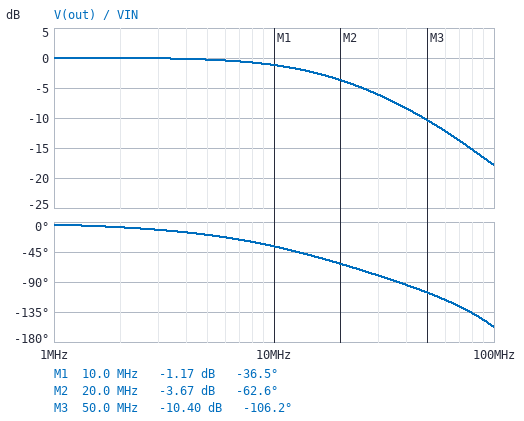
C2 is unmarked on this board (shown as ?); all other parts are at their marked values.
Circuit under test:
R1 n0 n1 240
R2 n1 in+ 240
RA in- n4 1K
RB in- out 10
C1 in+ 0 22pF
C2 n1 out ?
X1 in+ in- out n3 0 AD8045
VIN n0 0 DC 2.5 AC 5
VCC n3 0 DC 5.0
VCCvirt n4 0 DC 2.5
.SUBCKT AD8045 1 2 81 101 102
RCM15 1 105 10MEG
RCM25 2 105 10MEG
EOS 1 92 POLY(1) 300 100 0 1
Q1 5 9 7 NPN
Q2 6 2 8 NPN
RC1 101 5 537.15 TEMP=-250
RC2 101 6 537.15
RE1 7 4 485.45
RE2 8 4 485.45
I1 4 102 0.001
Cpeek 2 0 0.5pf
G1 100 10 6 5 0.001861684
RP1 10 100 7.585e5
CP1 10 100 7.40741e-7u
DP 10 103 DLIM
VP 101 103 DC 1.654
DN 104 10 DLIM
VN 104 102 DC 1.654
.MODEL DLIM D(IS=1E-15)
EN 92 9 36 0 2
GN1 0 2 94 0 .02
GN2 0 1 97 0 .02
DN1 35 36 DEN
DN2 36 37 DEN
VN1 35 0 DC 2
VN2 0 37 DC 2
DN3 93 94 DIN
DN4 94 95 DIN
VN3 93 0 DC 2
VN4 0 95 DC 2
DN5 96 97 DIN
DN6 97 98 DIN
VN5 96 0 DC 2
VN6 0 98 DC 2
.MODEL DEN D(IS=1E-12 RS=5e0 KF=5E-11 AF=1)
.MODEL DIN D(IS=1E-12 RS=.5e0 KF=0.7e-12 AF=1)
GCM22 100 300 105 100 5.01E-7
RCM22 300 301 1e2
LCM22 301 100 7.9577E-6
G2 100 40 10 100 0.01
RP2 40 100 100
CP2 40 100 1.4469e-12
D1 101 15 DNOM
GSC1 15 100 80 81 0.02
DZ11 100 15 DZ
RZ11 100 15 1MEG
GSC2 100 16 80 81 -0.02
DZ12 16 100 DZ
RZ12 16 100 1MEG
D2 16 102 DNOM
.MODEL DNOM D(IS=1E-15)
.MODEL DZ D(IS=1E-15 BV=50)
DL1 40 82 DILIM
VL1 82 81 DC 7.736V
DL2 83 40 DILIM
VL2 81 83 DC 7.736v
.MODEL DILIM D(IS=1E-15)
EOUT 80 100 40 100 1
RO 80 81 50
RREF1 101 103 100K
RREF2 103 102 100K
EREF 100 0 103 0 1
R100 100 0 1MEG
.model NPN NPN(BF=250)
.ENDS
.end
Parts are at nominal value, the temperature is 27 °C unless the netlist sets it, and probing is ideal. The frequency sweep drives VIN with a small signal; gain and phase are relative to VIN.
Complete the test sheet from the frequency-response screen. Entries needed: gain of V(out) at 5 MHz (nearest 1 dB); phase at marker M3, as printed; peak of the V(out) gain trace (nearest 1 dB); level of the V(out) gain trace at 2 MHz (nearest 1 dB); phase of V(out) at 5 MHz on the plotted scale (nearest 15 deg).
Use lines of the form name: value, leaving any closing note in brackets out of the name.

gain of V(out) at 5 MHz: 0 dB
phase at marker M3, as printed: -106.2 deg
peak of the V(out) gain trace: 0 dB
level of the V(out) gain trace at 2 MHz: 0 dB
phase of V(out) at 5 MHz on the plotted scale: -15 deg
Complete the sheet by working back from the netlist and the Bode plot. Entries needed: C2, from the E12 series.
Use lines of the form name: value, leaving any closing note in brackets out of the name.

C2, from the E12 series: 10 pF
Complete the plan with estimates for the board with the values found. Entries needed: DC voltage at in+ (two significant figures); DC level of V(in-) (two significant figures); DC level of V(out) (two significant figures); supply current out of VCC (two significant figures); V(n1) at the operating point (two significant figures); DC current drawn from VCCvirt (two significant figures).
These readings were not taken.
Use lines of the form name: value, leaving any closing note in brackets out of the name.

DC voltage at in+: 2.5 V
DC level of V(in-): 2.5 V
DC level of V(out): 2.5 V
supply current out of VCC: 1.0 mA
V(n1) at the operating point: 2.5 V
DC current drawn from VCCvirt: 310 nA
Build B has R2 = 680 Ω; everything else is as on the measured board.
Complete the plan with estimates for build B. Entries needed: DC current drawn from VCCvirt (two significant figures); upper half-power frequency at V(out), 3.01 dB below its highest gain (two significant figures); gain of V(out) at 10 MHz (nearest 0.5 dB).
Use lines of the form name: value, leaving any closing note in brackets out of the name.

DC current drawn from VCCvirt: 1.2 µA
upper half-power frequency at V(out), 3.01 dB below its highest gain: 8.6 MHz
gain of V(out) at 10 MHz: -3.5 dB
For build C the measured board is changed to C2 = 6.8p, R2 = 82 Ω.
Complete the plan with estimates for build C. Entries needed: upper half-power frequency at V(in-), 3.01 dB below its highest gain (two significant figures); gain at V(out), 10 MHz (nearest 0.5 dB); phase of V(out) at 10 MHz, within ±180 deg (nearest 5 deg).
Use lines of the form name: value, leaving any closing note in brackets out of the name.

upper half-power frequency at V(in-), 3.01 dB below its highest gain: 24 MHz
gain at V(out), 10 MHz: -0.5 dB
phase of V(out) at 10 MHz, within ±180 deg: -25 deg
